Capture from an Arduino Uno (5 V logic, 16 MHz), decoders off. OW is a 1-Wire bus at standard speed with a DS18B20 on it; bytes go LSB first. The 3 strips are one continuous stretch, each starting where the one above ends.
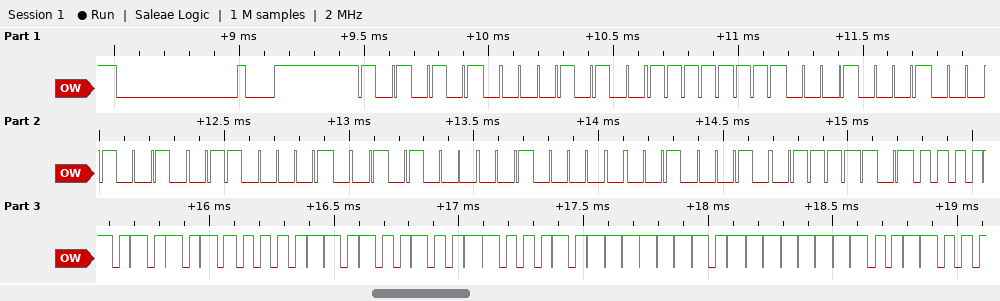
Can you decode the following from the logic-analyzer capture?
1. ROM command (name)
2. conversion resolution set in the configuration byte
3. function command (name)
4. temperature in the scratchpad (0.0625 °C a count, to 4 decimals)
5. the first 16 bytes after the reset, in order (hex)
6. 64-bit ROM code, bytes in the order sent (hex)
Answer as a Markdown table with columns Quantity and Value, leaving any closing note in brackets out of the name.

| Quantity | Value |
|---|---|
| ROM command | Match ROM |
| conversion resolution set in the configuration byte | 12 bits |
| function command | Read Scratchpad |
| temperature in the scratchpad | 85.0000 °C |
| the first 16 bytes after the reset, in order | 55 28 FF 88 48 86 14 04 44 BE 50 05 4B 46 7F FF |
| 64-bit ROM code, bytes in the order sent | 28 FF 88 48 86 14 04 44 |
